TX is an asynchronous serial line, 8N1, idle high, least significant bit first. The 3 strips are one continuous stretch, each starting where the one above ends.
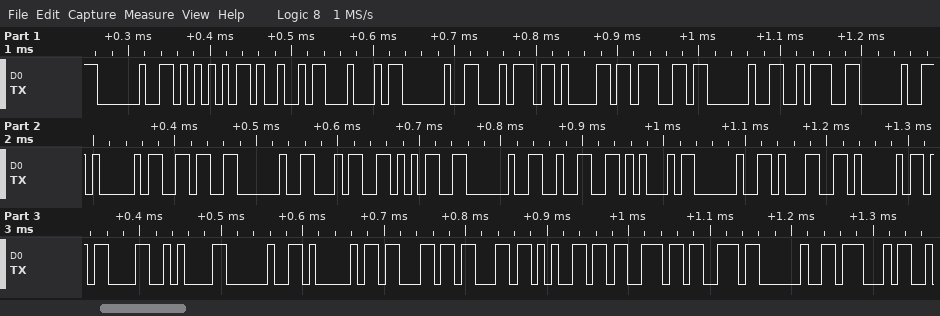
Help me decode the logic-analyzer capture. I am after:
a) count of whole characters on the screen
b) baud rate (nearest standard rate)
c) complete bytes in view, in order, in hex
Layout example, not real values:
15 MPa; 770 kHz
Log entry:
33; 115200 baud; 0x20 0x55 0x49 0x44 0x20 0x74 0x61 0x67 0x20 0x3A 0x20 0x41 0x36 0x20 0x34 0x35 0x20 0x32 0x45 0x20 0x31 0x41 0x0D 0x0A 0x20 0x41 0x63 0x63 0x65 0x73 0x73 0x20 0x47
